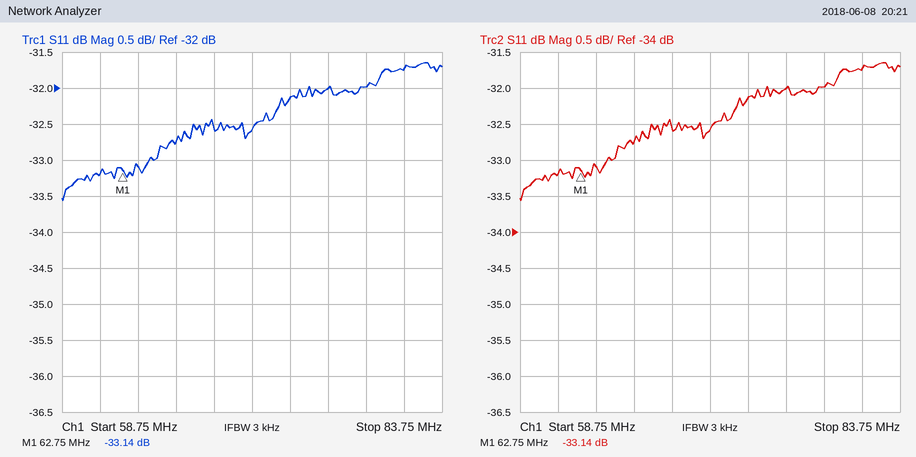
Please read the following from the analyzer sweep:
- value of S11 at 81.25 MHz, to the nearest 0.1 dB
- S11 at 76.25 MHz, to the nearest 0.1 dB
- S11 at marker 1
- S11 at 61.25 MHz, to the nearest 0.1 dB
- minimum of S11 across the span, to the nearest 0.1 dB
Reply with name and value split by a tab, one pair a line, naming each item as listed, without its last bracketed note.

value of S11 at 81.25 MHz, to the nearest 0.1 dB	-31.7 dB
S11 at 76.25 MHz, to the nearest 0.1 dB	-32.0 dB
S11 at marker 1	-33.14 dB
S11 at 61.25 MHz, to the nearest 0.1 dB	-33.2 dB
minimum of S11 across the span, to the nearest 0.1 dB	-33.6 dB
